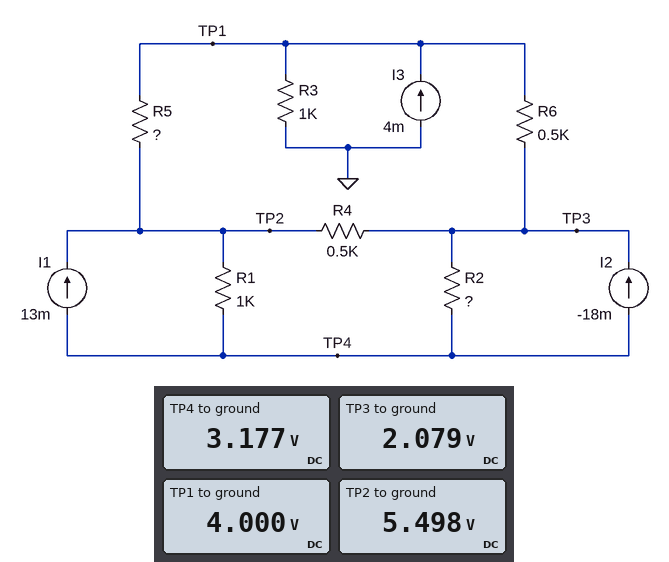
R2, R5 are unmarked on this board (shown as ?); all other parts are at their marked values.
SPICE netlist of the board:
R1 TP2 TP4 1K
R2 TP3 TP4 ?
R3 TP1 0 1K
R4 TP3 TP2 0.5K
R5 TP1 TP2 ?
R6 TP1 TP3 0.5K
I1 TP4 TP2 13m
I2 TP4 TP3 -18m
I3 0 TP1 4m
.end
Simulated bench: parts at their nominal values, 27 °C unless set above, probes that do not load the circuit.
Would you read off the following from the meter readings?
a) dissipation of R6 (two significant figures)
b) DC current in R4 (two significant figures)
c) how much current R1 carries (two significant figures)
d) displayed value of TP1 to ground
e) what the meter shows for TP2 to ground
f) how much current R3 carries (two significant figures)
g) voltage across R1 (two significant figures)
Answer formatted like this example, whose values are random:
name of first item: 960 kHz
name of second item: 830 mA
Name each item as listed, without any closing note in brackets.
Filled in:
dissipation of R6: 7.4 mW
DC current in R4: 6.8 mA
how much current R1 carries: 2.3 mA
displayed value of TP1 to ground: 4.000 V
what the meter shows for TP2 to ground: 5.498 V
how much current R3 carries: 4.0 mA
voltage across R1: 2.3 V
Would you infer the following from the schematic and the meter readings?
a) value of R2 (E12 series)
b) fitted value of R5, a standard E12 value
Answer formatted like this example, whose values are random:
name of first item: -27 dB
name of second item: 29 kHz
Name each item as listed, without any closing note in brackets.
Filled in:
value of R2: 150 Ω
fitted value of R5, a standard E12 value: 390 Ω
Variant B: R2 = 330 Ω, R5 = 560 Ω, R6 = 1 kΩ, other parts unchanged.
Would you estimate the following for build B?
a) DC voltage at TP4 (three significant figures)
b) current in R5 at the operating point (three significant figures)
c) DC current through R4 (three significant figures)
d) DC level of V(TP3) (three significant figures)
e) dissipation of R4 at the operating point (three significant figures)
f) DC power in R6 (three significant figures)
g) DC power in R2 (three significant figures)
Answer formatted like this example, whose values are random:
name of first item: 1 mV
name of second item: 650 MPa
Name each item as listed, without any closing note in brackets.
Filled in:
DC voltage at TP4: 3.59 V
current in R5 at the operating point: 2.69 mA
DC current through R4: 8.39 mA
DC level of V(TP3): 1.31 V
dissipation of R4 at the operating point: 35.2 mW
DC power in R6: 7.24 mW
DC power in R2: 15.8 mW
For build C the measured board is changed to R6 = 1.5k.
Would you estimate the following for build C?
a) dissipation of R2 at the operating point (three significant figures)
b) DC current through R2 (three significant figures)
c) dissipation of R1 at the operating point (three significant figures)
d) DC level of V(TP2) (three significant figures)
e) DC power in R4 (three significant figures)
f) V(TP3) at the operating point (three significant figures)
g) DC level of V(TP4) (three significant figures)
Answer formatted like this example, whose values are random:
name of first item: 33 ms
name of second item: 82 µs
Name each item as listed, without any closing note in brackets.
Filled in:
dissipation of R2 at the operating point: 9.22 mW
DC current through R2: 7.84 mA
dissipation of R1 at the operating point: 8.07 mW
DC level of V(TP2): 4.83 V
DC power in R4: 32.3 mW
V(TP3) at the operating point: 812 mV
DC level of V(TP4): 1.99 V
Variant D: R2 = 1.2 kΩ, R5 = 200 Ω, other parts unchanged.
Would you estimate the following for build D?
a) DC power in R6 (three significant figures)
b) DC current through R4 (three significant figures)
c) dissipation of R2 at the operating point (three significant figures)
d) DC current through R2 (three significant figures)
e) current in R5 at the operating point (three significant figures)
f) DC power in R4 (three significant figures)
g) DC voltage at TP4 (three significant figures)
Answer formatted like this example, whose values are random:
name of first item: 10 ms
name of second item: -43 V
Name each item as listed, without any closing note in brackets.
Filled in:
DC power in R6: 16.7 mW
DC current through R4: 8.10 mA
dissipation of R2 at the operating point: 20.3 mW
DC current through R2: 4.11 mA
current in R5 at the operating point: 5.79 mA
DC power in R4: 32.8 mW
DC voltage at TP4: 6.04 V
